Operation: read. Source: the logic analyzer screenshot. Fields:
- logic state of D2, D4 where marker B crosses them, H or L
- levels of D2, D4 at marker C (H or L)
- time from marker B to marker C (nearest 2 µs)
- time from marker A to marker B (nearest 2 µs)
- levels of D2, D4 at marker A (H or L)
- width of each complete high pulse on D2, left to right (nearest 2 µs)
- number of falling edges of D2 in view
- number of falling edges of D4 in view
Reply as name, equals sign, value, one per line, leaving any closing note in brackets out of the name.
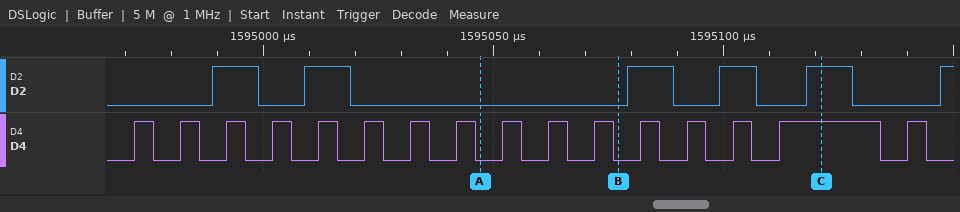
logic state of D2, D4 where marker B crosses them, H or L = D2=L, D4=L
levels of D2, D4 at marker C = D2=H, D4=H
time from marker B to marker C = 44 µs
time from marker A to marker B = 30 µs
levels of D2, D4 at marker A = D2=L, D4=L
width of each complete high pulse on D2, left to right = 10 µs, 10 µs, 10 µs, 8 µs, 10 µs
number of falling edges of D2 in view = 5
number of falling edges of D4 in view = 16
